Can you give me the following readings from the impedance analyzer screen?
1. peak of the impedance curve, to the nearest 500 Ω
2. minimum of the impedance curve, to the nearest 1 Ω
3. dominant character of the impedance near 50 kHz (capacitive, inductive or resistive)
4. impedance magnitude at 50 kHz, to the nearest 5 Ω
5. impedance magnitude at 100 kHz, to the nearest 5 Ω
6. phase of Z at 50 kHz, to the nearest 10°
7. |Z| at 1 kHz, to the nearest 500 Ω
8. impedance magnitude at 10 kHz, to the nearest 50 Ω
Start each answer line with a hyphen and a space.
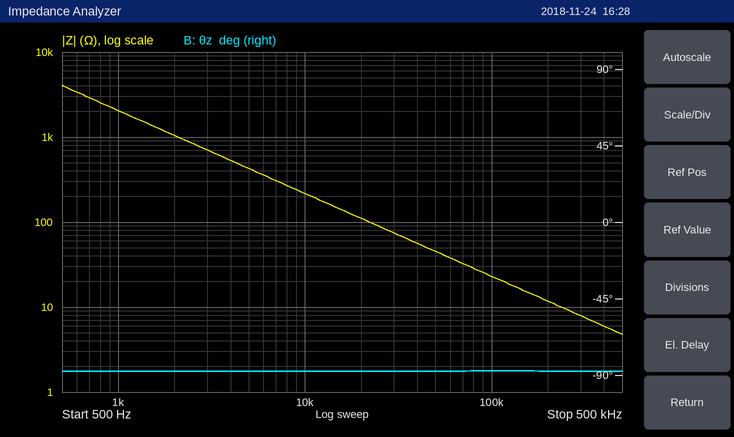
- 4.0 kΩ
- 5 Ω
- capacitive
- 45 Ω
- 25 Ω
- -90°
- 2.0 kΩ
- 200 Ω
